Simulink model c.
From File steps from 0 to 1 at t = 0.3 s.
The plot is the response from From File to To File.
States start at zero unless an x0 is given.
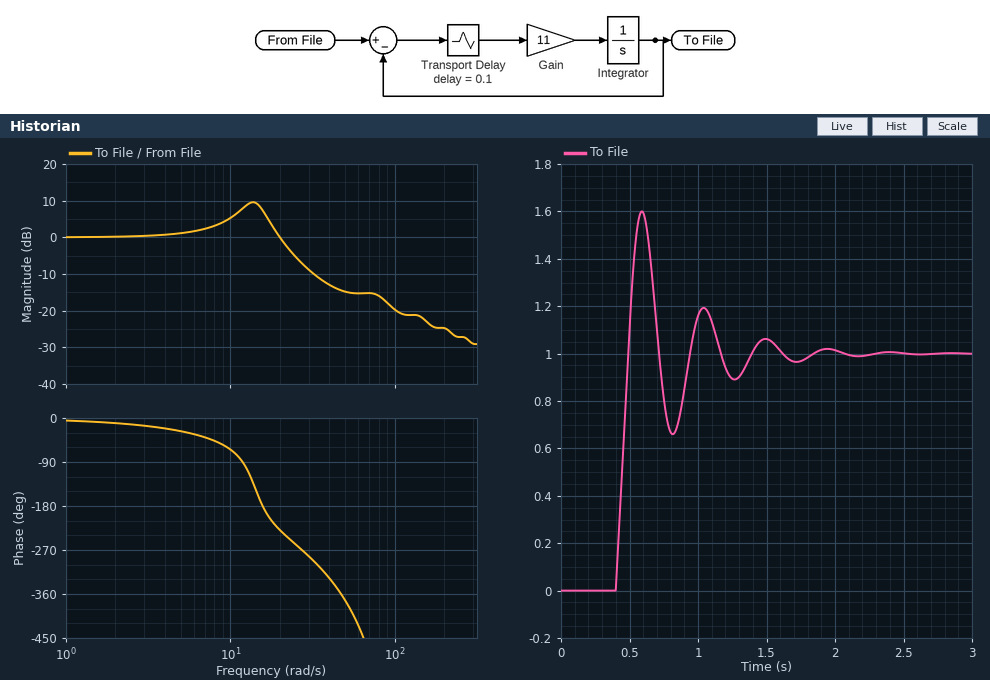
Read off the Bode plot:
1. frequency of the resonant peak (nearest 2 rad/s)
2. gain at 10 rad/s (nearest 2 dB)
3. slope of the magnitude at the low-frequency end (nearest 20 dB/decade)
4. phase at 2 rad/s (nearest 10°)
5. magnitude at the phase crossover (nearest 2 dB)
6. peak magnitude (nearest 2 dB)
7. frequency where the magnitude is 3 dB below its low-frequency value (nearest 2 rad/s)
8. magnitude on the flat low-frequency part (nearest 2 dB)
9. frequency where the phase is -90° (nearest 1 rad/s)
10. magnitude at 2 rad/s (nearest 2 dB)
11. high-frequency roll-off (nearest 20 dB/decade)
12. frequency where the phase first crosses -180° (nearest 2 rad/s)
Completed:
14 rad/s
6 dB
0 dB/decade
-10°
8 dB
10 dB
22 rad/s
0 dB
12 rad/s
0 dB
-20 dB/decade
16 rad/s
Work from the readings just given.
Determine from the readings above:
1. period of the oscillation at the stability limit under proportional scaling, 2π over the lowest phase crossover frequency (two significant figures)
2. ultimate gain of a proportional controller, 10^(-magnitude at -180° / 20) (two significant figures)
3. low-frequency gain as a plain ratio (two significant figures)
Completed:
0.39 s
0.40
1.0
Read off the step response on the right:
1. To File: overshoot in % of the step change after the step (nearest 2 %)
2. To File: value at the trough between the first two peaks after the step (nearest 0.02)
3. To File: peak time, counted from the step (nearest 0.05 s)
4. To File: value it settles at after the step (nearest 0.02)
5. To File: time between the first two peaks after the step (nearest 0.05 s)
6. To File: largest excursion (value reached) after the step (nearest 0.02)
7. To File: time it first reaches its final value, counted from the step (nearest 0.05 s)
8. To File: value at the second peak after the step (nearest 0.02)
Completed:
60 %
0.66
0.30 s
1.00
0.45 s
1.60
0.20 s
1.20
